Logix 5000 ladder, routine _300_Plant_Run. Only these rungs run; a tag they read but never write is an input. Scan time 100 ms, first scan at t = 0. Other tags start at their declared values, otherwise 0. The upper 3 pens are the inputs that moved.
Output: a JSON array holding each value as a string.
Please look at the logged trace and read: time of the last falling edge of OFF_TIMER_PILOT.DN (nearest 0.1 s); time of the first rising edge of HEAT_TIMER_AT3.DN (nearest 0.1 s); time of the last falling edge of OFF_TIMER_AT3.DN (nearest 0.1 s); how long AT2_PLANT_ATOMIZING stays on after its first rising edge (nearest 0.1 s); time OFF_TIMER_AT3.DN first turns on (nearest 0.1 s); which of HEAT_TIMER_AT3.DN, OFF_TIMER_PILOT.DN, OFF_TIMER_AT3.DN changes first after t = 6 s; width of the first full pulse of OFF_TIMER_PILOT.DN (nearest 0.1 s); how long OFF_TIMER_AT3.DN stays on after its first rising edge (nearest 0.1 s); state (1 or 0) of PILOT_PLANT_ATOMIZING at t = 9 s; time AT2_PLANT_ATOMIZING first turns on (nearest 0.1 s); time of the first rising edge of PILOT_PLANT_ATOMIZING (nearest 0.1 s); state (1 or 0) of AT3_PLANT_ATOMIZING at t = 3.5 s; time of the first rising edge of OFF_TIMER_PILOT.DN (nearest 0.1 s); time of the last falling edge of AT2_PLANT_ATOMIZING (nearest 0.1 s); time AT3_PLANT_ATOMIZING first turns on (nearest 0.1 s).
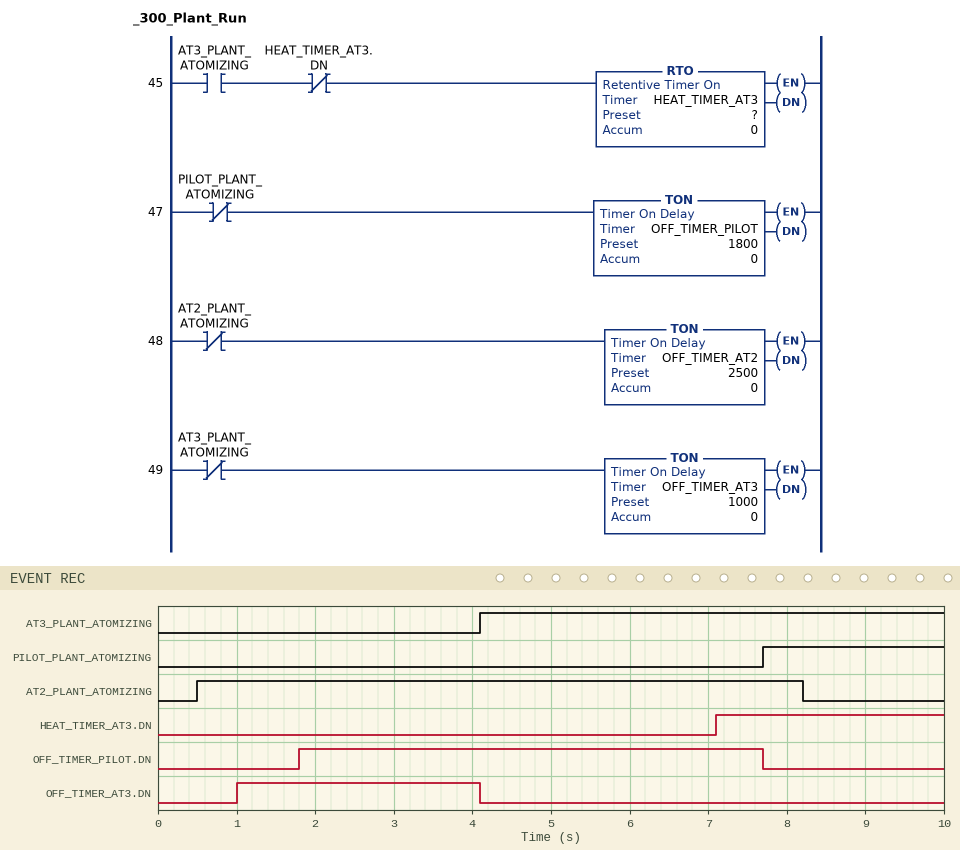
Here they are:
["7.7 s", "7.1 s", "4.1 s", "7.7 s", "1.0 s", "HEAT_TIMER_AT3.DN", "5.9 s", "3.1 s", "1", "0.5 s", "7.7 s", "0", "1.8 s", "8.2 s", "4.1 s"]
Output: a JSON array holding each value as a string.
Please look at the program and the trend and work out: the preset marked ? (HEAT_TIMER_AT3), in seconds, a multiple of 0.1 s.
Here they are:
["3.0 s"]
